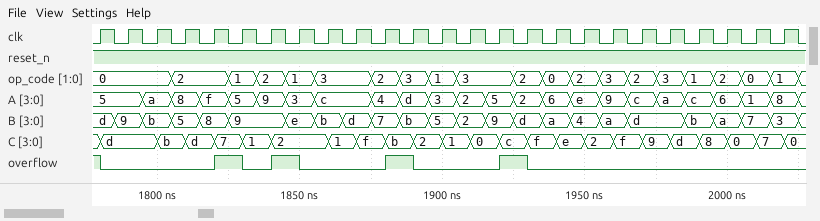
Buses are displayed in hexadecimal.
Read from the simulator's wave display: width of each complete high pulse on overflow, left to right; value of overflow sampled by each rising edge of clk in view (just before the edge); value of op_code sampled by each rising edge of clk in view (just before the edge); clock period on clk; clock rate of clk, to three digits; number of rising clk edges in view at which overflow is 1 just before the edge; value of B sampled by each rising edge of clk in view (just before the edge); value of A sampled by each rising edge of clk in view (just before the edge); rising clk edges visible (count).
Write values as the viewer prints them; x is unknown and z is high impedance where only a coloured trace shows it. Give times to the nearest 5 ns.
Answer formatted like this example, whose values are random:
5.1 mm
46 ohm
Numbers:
10 ns, 10 ns, 10 ns, 10 ns
1 0 0 0 0 1 0 1 0 0 0 1 0 0 0 1 0 0 0 0 0 0 0 0 0
0, 0, 0, 2, 2, 1, 2, 1, 3, 3, 2, 3, 1, 3, 3, 2, 0, 2, 3, 2, 3, 1, 2, 0, 1
10 ns
100 MHz
5
d, 9, b, 5, 8, 9, 9, e, b, d, 7, b, 5, 2, 9, d, a, 4, a, d, d, b, a, 7, 3
5, 5, a, 8, f, 5, 9, 3, c, c, 4, d, 3, 2, 5, 2, 6, e, 9, c, a, c, 6, 1, 8
25
